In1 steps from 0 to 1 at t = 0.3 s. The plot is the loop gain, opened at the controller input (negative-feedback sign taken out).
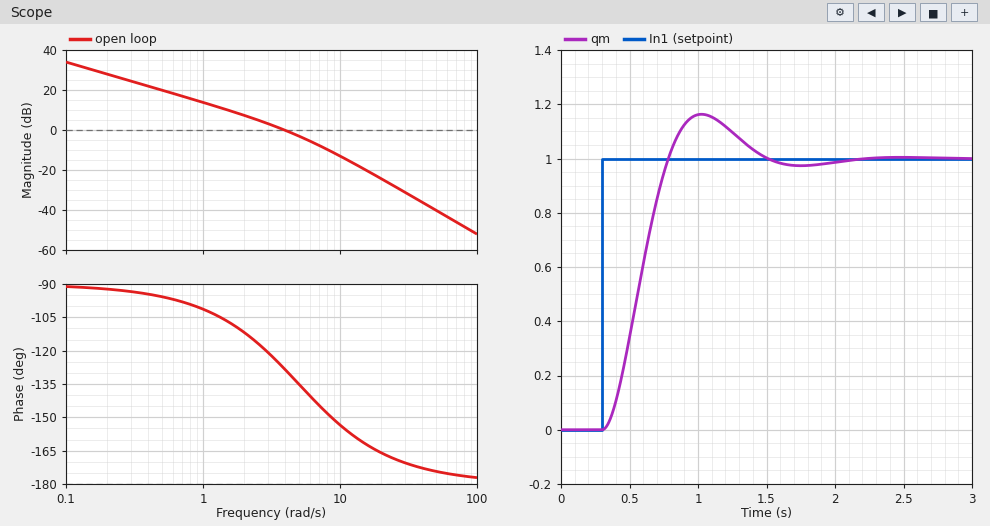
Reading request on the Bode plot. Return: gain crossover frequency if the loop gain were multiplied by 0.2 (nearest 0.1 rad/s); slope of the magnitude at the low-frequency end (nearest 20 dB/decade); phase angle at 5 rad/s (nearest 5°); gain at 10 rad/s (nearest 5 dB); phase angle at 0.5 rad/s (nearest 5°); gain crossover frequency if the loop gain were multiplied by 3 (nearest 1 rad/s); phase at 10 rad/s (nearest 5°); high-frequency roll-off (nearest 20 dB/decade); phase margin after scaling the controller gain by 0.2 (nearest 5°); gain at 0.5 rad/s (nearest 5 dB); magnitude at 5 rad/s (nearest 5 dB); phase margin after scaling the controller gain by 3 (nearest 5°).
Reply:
1.0 rad/s
-20 dB/decade
-135°
-15 dB
-95°
8 rad/s
-155°
-40 dB/decade
80°
20 dB
-5 dB
30°
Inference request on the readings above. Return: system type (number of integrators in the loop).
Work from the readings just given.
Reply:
1
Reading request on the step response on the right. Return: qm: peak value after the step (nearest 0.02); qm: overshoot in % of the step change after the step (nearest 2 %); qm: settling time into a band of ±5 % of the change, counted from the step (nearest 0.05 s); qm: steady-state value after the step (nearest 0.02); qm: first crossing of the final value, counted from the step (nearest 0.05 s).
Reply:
1.16
16 %
1.05 s
1.00
0.50 s
